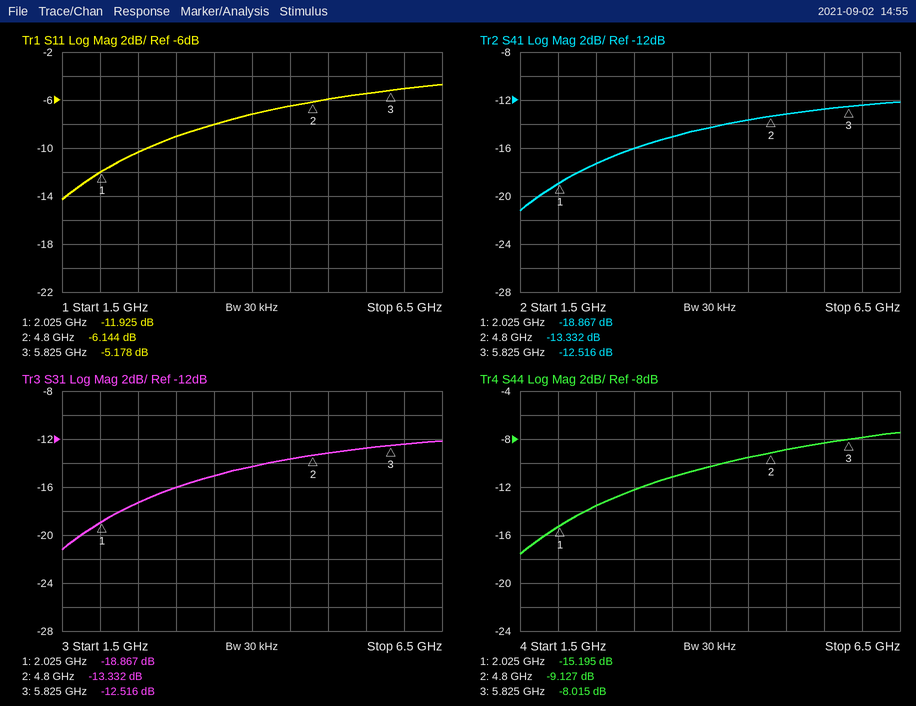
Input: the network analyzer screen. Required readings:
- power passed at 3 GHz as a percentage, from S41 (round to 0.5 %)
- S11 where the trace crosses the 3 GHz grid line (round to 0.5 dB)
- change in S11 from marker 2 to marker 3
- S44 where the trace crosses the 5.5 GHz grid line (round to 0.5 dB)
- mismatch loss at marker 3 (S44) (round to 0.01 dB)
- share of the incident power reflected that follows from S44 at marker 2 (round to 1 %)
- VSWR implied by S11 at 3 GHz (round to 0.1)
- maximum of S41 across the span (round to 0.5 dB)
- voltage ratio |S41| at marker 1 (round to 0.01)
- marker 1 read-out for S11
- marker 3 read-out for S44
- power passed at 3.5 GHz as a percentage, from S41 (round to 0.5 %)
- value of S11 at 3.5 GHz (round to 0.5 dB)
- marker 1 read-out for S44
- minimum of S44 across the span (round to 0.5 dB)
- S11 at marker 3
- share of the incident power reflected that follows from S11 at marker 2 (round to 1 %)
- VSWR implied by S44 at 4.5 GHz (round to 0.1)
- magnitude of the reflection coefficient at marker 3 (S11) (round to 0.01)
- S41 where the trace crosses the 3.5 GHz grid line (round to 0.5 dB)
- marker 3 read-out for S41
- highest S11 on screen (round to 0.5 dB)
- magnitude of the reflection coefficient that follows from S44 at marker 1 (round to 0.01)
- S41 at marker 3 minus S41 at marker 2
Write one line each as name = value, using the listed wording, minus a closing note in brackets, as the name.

power passed at 3 GHz as a percentage, from S41 = 2.5 %
S11 where the trace crosses the 3 GHz grid line = -9.0 dB
change in S11 from marker 2 to marker 3 = 0.966 dB
S44 where the trace crosses the 5.5 GHz grid line = -8.5 dB
mismatch loss at marker 3 (S44) = 0.75 dB
share of the incident power reflected that follows from S44 at marker 2 = 12 %
VSWR implied by S11 at 3 GHz = 2.1
maximum of S41 across the span = -12.0 dB
voltage ratio |S41| at marker 1 = 0.11
marker 1 read-out for S11 = -11.925 dB
marker 3 read-out for S44 = -8.015 dB
power passed at 3.5 GHz as a percentage, from S41 = 3.0 %
value of S11 at 3.5 GHz = -8.0 dB
marker 1 read-out for S44 = -15.195 dB
minimum of S44 across the span = -17.5 dB
S11 at marker 3 = -5.178 dB
share of the incident power reflected that follows from S11 at marker 2 = 24 %
VSWR implied by S44 at 4.5 GHz = 2.0
magnitude of the reflection coefficient at marker 3 (S11) = 0.55
S41 where the trace crosses the 3.5 GHz grid line = -15.0 dB
marker 3 read-out for S41 = -12.516 dB
highest S11 on screen = -4.5 dB
magnitude of the reflection coefficient that follows from S44 at marker 1 = 0.17
S41 at marker 3 minus S41 at marker 2 = 0.816 dB
